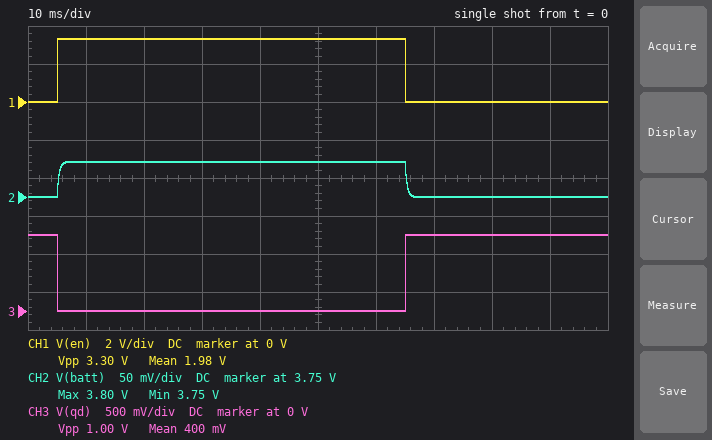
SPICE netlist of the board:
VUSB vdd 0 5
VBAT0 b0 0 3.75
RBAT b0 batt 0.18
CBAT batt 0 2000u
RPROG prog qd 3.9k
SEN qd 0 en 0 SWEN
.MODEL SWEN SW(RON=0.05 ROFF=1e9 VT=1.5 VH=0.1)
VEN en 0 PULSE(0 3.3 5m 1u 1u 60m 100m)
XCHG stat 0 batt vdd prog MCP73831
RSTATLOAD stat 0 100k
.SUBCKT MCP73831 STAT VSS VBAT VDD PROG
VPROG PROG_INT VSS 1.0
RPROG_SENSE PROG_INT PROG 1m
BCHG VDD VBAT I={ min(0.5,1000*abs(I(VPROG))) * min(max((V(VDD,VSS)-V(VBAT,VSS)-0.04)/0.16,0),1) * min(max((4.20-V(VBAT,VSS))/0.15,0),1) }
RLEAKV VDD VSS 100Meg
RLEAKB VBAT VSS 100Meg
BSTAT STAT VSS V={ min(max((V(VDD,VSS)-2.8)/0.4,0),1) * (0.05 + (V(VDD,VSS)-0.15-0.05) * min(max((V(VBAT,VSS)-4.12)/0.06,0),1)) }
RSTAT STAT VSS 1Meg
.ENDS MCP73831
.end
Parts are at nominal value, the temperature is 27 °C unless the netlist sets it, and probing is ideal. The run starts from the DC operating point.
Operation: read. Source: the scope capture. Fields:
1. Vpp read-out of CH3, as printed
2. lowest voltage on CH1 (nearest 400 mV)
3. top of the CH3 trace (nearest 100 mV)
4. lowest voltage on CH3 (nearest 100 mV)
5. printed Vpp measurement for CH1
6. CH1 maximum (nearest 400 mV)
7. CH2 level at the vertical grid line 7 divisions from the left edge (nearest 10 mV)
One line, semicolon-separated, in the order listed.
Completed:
1.00 V; 0 V; 1.0 V; 0 V; 3.30 V; 3.2 V; 3.75 V
